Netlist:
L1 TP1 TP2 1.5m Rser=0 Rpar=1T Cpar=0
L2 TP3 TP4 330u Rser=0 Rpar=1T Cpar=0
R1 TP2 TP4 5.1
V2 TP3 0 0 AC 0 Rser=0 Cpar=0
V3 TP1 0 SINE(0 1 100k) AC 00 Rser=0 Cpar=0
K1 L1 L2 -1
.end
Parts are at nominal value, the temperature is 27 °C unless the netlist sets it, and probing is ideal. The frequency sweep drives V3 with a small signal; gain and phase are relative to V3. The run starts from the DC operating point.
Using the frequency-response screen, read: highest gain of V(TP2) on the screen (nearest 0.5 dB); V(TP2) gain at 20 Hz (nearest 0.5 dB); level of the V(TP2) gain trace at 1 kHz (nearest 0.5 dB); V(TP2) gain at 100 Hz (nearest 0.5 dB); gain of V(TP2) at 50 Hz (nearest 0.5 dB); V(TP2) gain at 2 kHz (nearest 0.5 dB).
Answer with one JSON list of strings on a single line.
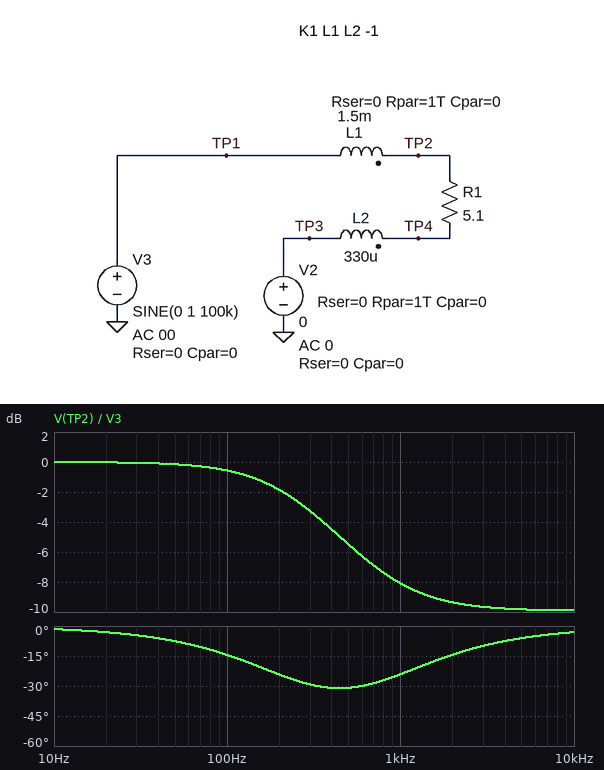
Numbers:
["0 dB", "0 dB", "-8.0 dB", "-0.5 dB", "0 dB", "-9.5 dB"]
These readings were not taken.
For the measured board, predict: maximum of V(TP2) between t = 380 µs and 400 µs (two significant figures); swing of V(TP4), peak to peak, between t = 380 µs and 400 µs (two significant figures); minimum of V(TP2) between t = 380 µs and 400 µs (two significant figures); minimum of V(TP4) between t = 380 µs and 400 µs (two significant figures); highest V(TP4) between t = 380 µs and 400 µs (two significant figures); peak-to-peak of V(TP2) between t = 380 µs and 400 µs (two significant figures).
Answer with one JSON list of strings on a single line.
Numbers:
["320 mV", "640 mV", "-320 mV", "-320 mV", "320 mV", "640 mV"]
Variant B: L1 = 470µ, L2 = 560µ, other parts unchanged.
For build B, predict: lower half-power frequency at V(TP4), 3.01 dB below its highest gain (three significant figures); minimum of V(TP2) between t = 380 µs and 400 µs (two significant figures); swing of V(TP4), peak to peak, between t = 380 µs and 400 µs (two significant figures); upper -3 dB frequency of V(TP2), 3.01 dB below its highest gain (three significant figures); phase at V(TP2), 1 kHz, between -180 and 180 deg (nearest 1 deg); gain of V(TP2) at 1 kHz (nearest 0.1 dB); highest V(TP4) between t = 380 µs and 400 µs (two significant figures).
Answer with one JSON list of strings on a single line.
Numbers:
["395 Hz", "-520 mV", "1.0 V", "585 Hz", "-16 deg", "-4.3 dB", "520 mV"]
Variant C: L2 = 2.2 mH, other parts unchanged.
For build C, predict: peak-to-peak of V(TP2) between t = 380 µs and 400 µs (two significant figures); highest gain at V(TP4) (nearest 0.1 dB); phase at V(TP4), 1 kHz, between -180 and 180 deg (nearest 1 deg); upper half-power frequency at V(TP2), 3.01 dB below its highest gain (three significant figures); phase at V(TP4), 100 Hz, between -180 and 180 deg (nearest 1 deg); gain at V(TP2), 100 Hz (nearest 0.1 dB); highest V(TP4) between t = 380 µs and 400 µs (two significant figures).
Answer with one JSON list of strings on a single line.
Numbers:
["1.1 V", "-5.2 dB", "6 deg", "175 Hz", "48 deg", "-1.6 dB", "550 mV"]
